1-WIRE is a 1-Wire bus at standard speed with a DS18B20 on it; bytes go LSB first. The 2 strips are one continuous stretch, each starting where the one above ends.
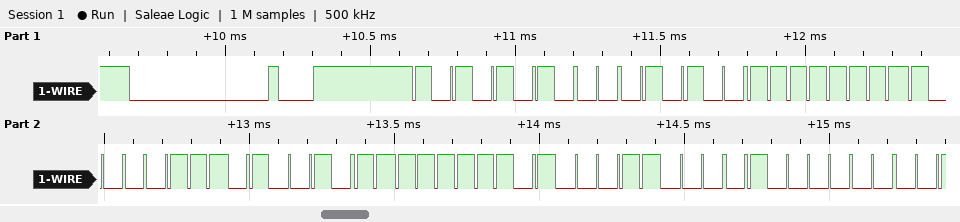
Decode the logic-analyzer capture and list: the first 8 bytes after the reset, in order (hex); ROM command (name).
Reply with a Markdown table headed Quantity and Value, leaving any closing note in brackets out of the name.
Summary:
| Quantity | Value |
|---|---|
| the first 8 bytes after the reset, in order | 55 28 FF E1 D2 BF 18 02 |
| ROM command | Match ROM |
